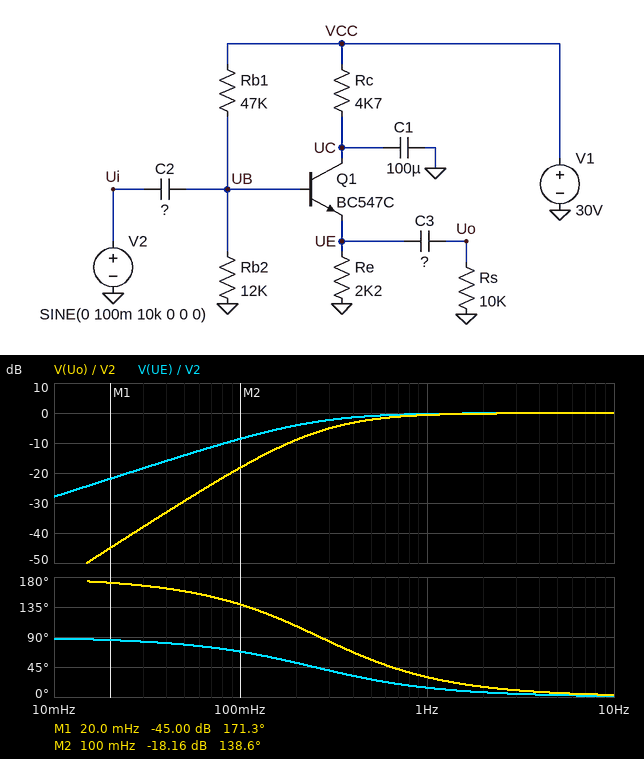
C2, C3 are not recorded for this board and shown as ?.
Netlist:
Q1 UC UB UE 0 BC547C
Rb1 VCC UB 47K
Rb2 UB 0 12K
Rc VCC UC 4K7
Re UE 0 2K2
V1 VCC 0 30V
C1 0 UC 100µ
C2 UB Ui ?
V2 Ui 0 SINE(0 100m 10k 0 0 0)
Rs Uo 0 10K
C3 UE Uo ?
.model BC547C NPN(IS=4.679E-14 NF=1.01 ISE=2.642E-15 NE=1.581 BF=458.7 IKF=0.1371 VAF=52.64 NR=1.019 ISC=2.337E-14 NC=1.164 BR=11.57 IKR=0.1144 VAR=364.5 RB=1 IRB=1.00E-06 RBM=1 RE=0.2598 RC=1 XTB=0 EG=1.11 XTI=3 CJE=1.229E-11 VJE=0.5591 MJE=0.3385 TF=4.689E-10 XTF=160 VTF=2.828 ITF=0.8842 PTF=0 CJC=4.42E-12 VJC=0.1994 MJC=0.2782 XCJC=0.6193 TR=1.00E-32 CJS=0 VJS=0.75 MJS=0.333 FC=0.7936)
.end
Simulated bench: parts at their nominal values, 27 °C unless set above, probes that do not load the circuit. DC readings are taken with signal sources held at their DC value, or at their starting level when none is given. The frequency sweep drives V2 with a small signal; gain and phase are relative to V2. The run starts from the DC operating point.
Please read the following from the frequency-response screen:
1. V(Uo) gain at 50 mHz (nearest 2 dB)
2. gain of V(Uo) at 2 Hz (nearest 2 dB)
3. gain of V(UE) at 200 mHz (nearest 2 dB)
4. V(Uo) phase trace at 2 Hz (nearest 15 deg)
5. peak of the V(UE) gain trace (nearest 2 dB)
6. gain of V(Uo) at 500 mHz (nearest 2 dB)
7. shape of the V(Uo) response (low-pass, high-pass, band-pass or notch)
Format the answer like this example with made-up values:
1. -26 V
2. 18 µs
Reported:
1. -30 dB
2. 0 dB
3. -4 dB
4. 15 deg
5. 0 dB
6. -2 dB
7. high-pass
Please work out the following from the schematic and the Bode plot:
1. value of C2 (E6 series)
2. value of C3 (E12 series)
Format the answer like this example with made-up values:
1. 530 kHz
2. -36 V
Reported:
1. 68 µF
2. 56 µF
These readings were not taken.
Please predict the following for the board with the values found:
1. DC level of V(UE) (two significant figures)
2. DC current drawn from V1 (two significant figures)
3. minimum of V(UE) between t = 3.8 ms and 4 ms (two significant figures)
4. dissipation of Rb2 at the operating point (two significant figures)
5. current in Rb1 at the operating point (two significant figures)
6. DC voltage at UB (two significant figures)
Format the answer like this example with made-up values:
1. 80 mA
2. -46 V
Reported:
1. 5.4 V
2. 3.0 mA
3. 5.3 V
4. 3.1 mW
5. 510 µA
6. 6.1 V
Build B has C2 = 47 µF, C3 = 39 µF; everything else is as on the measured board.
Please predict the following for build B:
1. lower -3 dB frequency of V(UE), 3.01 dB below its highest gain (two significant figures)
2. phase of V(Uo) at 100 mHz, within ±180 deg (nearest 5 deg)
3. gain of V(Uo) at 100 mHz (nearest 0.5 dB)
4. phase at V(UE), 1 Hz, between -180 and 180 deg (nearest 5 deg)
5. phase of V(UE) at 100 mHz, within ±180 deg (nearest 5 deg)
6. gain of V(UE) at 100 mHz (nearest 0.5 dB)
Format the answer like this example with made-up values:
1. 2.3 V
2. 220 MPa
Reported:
1. 360 mHz
2. 150 deg
3. -24.0 dB
4. 20 deg
5. 75 deg
6. -11.5 dB
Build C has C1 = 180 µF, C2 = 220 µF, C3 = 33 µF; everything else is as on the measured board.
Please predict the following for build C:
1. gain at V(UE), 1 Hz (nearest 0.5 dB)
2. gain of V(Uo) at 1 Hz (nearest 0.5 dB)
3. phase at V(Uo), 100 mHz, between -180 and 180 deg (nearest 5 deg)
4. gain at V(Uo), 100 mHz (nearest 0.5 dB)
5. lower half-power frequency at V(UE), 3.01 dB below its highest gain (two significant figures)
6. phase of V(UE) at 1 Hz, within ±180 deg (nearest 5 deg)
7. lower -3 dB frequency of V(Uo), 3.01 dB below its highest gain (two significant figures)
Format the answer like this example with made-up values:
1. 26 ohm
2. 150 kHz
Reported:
1. 0 dB
2. -1.0 dB
3. 115 deg
4. -16.0 dB
5. 76 mHz
6. 5 deg
7. 490 mHz
